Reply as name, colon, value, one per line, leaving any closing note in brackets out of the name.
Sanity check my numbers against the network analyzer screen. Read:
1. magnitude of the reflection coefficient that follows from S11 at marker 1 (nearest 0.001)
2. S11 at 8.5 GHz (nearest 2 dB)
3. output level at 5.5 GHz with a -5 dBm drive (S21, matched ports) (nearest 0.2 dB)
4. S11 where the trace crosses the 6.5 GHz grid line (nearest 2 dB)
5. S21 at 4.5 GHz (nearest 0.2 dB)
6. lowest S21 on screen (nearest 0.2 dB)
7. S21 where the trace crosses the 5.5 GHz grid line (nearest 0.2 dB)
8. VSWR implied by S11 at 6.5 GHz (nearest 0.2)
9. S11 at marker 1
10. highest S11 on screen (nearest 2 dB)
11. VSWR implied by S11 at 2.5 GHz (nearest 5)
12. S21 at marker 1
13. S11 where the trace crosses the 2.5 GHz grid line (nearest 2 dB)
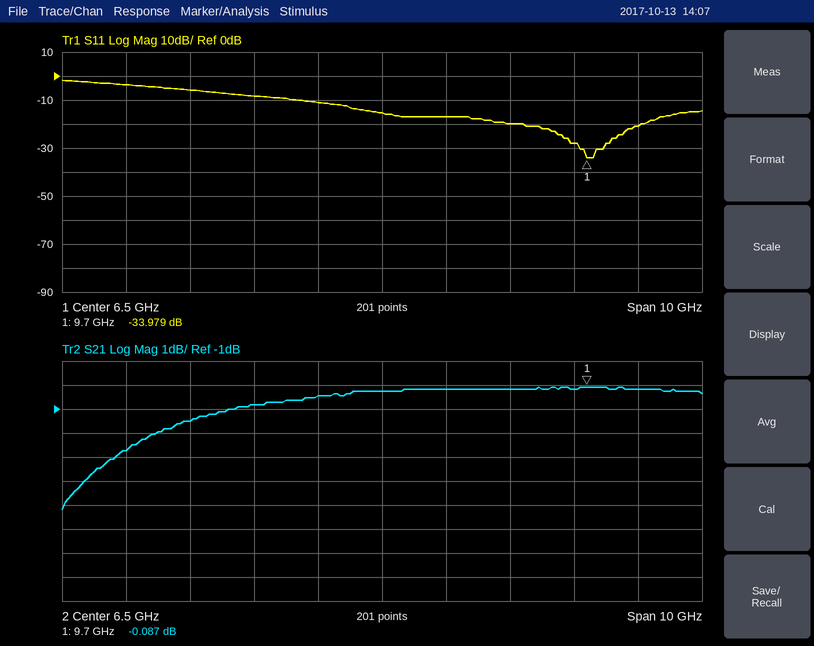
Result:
magnitude of the reflection coefficient that follows from S11 at marker 1: 0.020
S11 at 8.5 GHz: -20 dB
output level at 5.5 GHz with a -5 dBm drive (S21, matched ports): -5.4 dBm
S11 where the trace crosses the 6.5 GHz grid line: -16 dB
S21 at 4.5 GHz: -0.8 dB
lowest S21 on screen: -5.2 dB
S21 where the trace crosses the 5.5 GHz grid line: -0.4 dB
VSWR implied by S11 at 6.5 GHz: 1.4
S11 at marker 1: -33.979 dB
highest S11 on screen: -2 dB
VSWR implied by S11 at 2.5 GHz: 5
S21 at marker 1: -0.087 dB
S11 where the trace crosses the 2.5 GHz grid line: -4 dB
